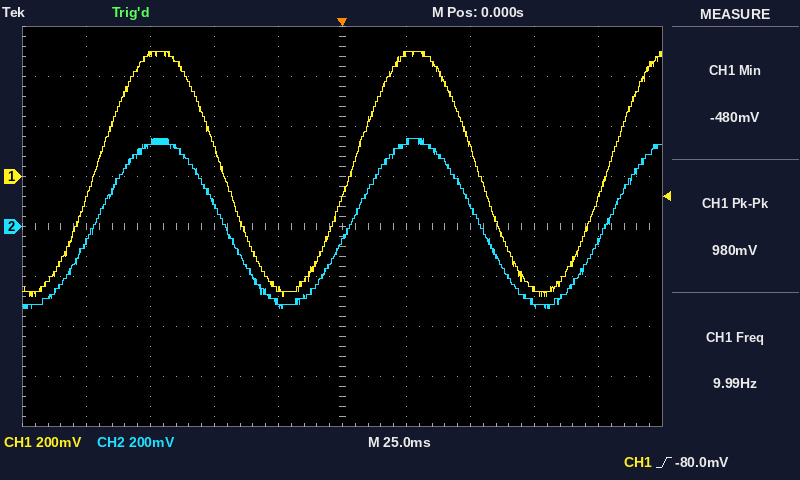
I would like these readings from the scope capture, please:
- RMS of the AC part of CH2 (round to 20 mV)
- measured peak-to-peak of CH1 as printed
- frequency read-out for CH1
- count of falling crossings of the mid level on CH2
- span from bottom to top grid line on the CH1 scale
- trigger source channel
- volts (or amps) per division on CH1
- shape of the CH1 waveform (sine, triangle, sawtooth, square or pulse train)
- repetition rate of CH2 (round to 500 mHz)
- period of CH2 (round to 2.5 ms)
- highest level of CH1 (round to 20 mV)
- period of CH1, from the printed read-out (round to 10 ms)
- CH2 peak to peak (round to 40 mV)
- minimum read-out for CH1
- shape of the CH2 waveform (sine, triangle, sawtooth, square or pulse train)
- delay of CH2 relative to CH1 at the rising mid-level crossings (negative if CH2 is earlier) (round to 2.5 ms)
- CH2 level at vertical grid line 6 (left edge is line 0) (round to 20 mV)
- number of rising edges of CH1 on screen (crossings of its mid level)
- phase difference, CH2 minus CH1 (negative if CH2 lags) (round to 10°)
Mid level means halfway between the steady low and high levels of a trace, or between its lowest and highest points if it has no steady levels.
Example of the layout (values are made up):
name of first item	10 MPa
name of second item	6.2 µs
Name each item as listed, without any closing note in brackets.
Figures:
RMS of the AC part of CH2	240 mV
measured peak-to-peak of CH1 as printed	980 mV
frequency read-out for CH1	9.99 Hz
count of falling crossings of the mid level on CH2	2
span from bottom to top grid line on the CH1 scale	1.6 V
trigger source channel	CH1
volts (or amps) per division on CH1	200 mV
shape of the CH1 waveform	sine
repetition rate of CH2	10.0 Hz
period of CH2	100.0 ms
highest level of CH1	500 mV
period of CH1, from the printed read-out	100 ms
CH2 peak to peak	680 mV
minimum read-out for CH1	-480 mV
shape of the CH2 waveform	sine
delay of CH2 relative to CH1 at the rising mid-level crossings (negative if CH2 is earlier)	0.0 ms
CH2 level at vertical grid line 6 (left edge is line 0)	340 mV
number of rising edges of CH1 on screen	3
phase difference, CH2 minus CH1 (negative if CH2 lags)	0°
